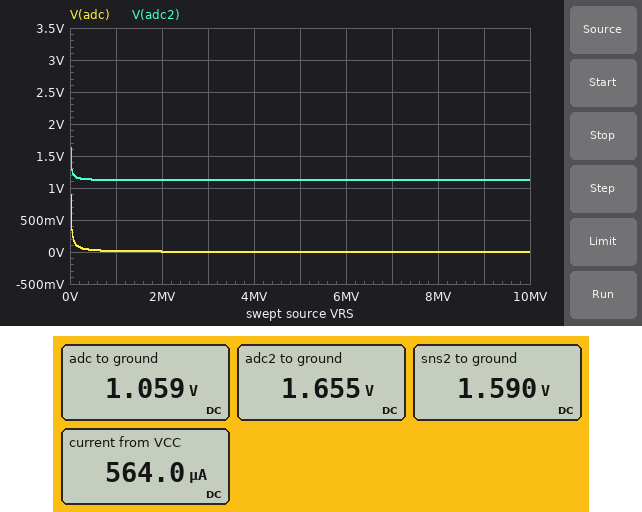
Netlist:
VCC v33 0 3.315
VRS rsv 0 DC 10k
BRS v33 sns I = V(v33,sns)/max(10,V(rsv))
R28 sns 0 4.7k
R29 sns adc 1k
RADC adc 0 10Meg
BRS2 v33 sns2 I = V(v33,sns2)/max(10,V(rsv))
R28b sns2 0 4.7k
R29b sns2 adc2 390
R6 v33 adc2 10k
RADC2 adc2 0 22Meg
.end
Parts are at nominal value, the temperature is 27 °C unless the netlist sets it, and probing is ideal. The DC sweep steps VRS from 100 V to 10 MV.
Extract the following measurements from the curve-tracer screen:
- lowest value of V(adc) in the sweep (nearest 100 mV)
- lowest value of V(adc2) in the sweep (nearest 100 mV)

0 V
1.1 V
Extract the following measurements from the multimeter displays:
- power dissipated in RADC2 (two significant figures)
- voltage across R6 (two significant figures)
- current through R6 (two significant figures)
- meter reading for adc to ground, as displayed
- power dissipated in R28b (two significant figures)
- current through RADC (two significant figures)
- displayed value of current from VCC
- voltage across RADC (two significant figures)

120 nW
1.7 V
170 µA
1.059 V
540 µW
110 nA
564.0 µA
1.1 V
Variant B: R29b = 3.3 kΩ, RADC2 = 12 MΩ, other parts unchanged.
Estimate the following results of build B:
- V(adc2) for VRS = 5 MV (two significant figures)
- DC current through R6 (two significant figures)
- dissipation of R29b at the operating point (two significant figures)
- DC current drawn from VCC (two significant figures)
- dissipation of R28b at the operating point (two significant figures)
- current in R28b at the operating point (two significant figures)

1.5 V
140 µA
62 µW
540 µA
480 µW
320 µA
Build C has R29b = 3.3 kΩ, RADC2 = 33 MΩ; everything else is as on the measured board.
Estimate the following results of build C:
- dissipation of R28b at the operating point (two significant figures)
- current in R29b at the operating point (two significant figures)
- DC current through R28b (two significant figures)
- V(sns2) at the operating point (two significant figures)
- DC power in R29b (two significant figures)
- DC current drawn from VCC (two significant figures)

480 µW
140 µA
320 µA
1.5 V
62 µW
540 µA
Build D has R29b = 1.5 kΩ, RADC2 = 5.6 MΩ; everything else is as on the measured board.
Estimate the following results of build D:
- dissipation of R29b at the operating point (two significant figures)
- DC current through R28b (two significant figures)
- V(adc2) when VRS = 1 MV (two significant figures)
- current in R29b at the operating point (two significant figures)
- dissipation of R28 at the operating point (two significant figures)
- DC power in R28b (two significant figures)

35 µW
330 µA
1.3 V
150 µA
240 µW
510 µW
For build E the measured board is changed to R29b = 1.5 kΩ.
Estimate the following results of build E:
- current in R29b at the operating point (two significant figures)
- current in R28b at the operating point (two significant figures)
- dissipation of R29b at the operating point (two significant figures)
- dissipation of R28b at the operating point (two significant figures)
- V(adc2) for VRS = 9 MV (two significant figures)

150 µA
330 µA
35 µW
510 µW
1.3 V
